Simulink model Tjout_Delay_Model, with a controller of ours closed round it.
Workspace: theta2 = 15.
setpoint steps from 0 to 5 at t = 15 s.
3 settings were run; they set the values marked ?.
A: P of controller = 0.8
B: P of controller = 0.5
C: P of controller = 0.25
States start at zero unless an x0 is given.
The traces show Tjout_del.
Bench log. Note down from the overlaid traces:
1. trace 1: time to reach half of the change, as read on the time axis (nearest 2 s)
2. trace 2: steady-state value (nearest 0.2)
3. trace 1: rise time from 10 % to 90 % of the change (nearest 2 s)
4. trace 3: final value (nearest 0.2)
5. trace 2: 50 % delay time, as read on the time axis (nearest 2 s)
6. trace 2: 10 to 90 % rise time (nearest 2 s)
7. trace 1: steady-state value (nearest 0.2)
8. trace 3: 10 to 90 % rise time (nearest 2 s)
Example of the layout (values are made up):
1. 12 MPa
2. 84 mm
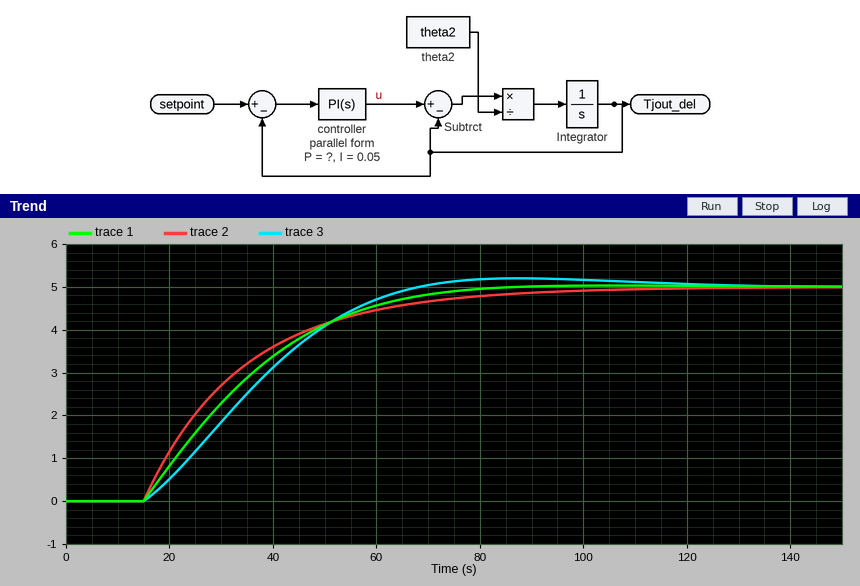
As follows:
1. 32 s
2. 5.0
3. 40 s
4. 5.0
5. 28 s
6. 44 s
7. 5.0
8. 36 s
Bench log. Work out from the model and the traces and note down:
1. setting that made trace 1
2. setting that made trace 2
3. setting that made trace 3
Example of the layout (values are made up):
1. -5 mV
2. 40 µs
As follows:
1. B
2. A
3. C
